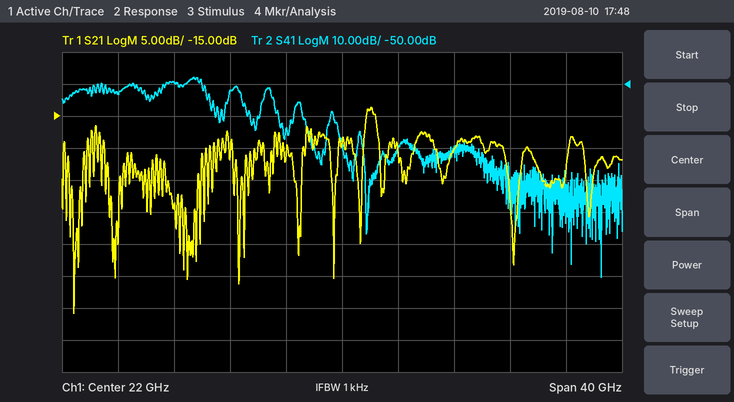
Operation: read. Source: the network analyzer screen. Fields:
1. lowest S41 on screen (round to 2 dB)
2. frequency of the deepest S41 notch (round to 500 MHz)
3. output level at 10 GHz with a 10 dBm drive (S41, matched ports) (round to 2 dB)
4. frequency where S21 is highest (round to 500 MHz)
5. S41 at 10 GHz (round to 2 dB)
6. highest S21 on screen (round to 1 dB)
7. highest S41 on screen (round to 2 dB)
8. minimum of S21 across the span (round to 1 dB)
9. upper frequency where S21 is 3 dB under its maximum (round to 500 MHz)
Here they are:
-110 dB
40.5 GHz
-40 dBm
24.0 GHz
-50 dB
-14 dB
-48 dB
-46 dB
24.5 GHz
